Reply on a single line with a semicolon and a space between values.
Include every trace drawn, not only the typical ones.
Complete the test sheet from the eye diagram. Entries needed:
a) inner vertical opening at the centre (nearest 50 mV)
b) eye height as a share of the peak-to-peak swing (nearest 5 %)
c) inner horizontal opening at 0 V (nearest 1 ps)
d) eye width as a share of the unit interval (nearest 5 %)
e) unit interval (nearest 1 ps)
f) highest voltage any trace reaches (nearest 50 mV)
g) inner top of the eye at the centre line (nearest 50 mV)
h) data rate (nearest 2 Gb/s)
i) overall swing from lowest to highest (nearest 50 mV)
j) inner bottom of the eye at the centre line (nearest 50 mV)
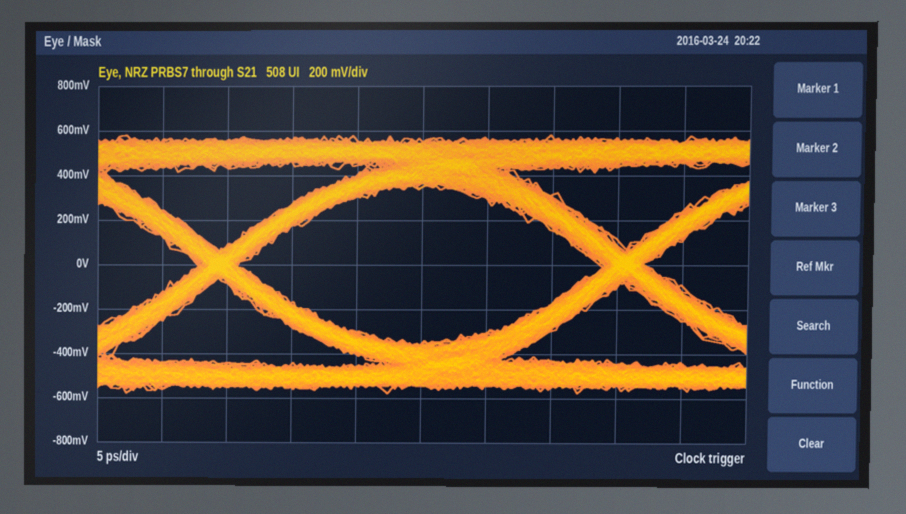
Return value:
700 mV; 60 %; 28 ps; 90 %; 31 ps; 600 mV; 350 mV; 32 Gb/s; 1.15 V; -350 mV
